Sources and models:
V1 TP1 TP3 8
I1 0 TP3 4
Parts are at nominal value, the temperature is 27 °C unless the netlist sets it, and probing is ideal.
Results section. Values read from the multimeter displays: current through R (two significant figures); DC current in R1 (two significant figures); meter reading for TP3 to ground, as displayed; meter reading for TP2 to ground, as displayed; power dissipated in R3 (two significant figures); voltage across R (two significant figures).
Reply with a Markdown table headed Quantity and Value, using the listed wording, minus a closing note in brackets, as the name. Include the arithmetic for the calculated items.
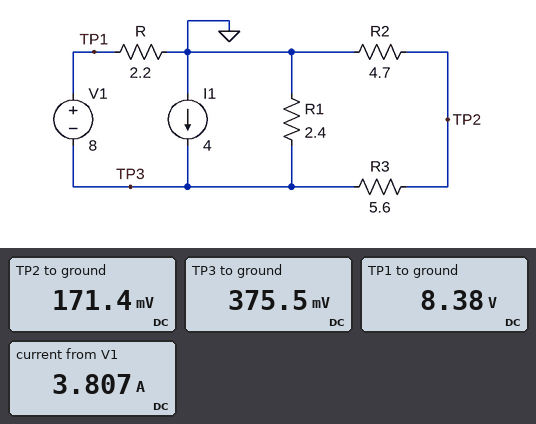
| Quantity | Value |
|---|---|
| current through R | (8.38 V) / 2.2 Ω = 3.8 A |
| DC current in R1 | (375.5 mV) / 2.4 Ω = 160 mA |
| meter reading for TP3 to ground, as displayed | 375.5 mV |
| meter reading for TP2 to ground, as displayed | 171.4 mV |
| power dissipated in R3 | (375.5 mV - 171.4 mV)^2 / 5.6 Ω = 7.4 mW |
| voltage across R | 8.38 V = 8.4 V |
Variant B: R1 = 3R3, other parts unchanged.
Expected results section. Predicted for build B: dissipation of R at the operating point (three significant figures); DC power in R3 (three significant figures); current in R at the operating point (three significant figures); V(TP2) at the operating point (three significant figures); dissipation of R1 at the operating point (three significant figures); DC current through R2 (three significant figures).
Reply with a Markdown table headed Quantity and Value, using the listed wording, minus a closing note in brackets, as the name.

| Quantity | Value |
|---|---|
| dissipation of R at the operating point | 32.3 W |
| DC power in R3 | 9.56 mW |
| current in R at the operating point | 3.83 A |
| V(TP2) at the operating point | 194 mV |
| dissipation of R1 at the operating point | 54.9 mW |
| DC current through R2 | 41.3 mA |
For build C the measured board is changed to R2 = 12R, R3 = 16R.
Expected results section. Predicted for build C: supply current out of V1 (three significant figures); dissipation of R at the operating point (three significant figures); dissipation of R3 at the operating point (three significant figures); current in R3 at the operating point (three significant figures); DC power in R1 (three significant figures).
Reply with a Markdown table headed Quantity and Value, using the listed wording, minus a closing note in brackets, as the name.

| Quantity | Value |
|---|---|
| supply current out of V1 | 3.82 A |
| dissipation of R at the operating point | 32.1 W |
| dissipation of R3 at the operating point | 3.28 mW |
| current in R3 at the operating point | 14.3 mA |
| DC power in R1 | 67.0 mW |
